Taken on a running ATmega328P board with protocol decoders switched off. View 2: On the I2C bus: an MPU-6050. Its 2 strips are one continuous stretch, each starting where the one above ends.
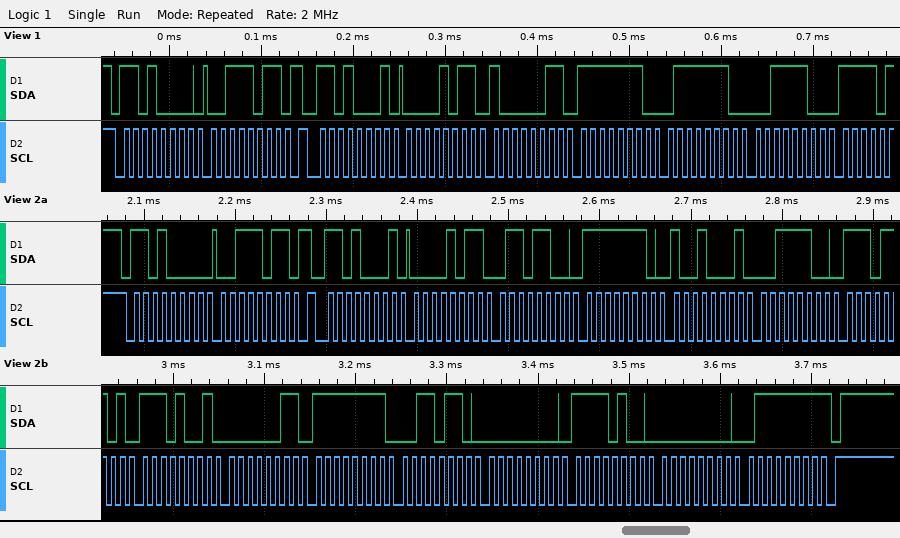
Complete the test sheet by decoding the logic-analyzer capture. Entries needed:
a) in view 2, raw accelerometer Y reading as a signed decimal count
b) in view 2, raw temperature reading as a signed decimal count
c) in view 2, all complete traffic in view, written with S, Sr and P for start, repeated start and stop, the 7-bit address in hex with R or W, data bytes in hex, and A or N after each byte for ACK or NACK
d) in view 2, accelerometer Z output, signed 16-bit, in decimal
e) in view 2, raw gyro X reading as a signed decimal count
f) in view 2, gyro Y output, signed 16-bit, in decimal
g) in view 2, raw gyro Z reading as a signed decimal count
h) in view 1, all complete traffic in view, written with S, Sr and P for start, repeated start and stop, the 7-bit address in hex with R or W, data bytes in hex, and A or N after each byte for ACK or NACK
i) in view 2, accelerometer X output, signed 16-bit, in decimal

-367
-5885
S 68W A 3B A Sr 68R A 0B A 6C A FE A 91 A 3C A ED A E9 A 03 A FF A 36 A 00 A F4 A 00 A 7F N P
15597
-202
244
127
S 68W A 3B A Sr 68R A 0B A 83 A FE A 7E A 3C A
2924
